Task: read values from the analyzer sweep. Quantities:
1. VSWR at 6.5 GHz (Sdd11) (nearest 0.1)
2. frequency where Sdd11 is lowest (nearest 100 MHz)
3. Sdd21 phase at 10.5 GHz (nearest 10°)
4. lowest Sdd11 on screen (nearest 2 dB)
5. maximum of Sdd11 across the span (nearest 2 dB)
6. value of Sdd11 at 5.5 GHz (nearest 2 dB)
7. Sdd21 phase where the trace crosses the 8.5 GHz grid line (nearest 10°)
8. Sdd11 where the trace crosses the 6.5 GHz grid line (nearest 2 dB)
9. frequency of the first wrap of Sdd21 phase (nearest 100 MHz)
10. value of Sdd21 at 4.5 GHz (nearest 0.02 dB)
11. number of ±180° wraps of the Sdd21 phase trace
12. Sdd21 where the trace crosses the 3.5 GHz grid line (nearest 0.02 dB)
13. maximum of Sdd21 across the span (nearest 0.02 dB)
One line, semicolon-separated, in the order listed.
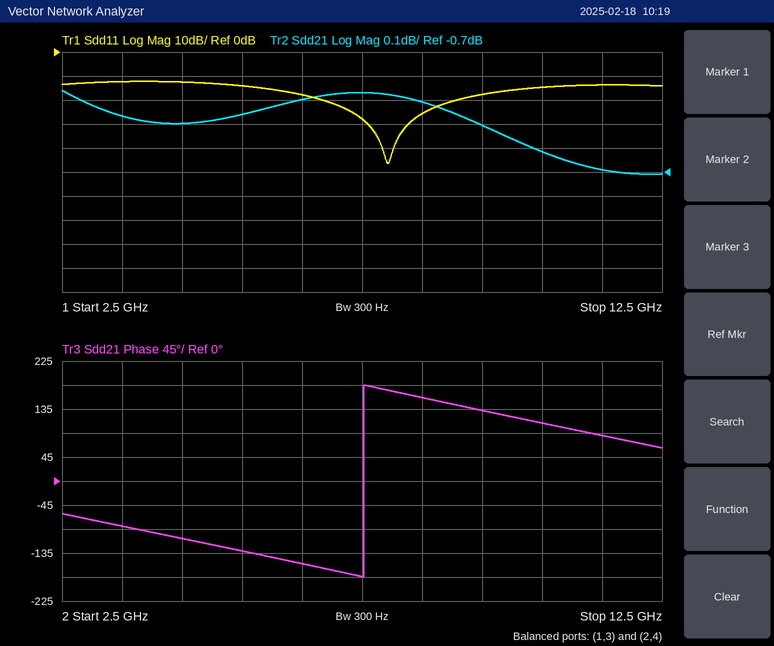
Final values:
1.3; 7.9 GHz; 110°; -46 dB; -12 dB; -14 dB; 160°; -18 dB; 7.5 GHz; -0.50 dB; 1; -0.46 dB; -0.36 dB
